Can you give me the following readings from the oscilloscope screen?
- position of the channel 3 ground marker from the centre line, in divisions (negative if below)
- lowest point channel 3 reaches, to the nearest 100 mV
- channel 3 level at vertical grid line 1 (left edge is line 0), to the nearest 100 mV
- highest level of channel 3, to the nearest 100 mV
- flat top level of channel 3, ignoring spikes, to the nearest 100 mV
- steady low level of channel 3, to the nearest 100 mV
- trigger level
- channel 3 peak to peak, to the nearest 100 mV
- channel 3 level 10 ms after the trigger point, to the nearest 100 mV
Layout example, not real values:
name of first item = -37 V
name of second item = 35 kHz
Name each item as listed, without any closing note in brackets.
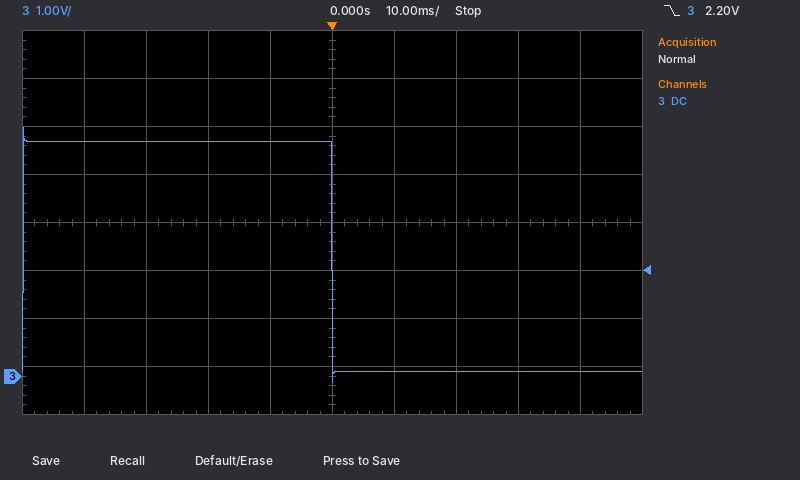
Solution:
position of the channel 3 ground marker from the centre line, in divisions = -3.2 div
lowest point channel 3 reaches, to the nearest 100 mV = -100 mV
channel 3 level at vertical grid line 1 (left edge is line 0), to the nearest 100 mV = 4.9 V
highest level of channel 3, to the nearest 100 mV = 5.2 V
flat top level of channel 3, ignoring spikes, to the nearest 100 mV = 4.9 V
steady low level of channel 3, to the nearest 100 mV = 100 mV
trigger level = 2.20 V
channel 3 peak to peak, to the nearest 100 mV = 5.3 V
channel 3 level 10 ms after the trigger point, to the nearest 100 mV = 100 mV
